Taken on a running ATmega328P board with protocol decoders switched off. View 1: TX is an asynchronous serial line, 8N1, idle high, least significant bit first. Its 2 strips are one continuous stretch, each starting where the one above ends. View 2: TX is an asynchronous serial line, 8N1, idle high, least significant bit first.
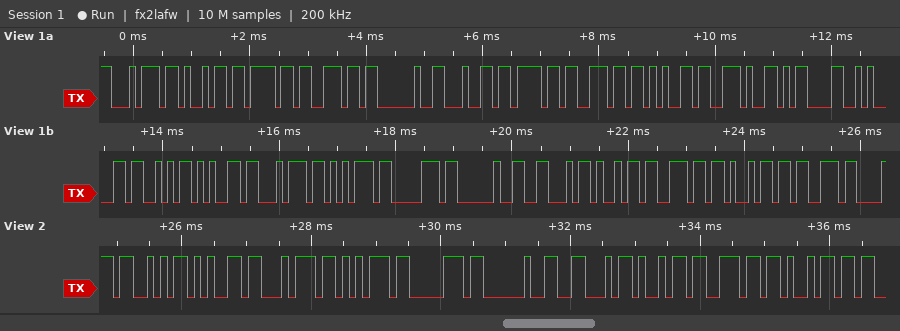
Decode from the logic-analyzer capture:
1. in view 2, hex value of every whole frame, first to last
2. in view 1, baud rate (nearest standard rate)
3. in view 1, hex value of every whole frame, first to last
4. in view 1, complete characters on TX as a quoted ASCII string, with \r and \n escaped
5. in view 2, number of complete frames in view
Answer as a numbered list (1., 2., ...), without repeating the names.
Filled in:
1. 53 65 74 75 70 20 46 69 6E 69
2. 9600 baud
3. 74 69 6F 6E 20 64 6F 6E 65 2E 0D 0A 53 65 74 75 70 20 46 69 6E 69 73
4. "tion done.\r\nSetup Finis"
5. 10
